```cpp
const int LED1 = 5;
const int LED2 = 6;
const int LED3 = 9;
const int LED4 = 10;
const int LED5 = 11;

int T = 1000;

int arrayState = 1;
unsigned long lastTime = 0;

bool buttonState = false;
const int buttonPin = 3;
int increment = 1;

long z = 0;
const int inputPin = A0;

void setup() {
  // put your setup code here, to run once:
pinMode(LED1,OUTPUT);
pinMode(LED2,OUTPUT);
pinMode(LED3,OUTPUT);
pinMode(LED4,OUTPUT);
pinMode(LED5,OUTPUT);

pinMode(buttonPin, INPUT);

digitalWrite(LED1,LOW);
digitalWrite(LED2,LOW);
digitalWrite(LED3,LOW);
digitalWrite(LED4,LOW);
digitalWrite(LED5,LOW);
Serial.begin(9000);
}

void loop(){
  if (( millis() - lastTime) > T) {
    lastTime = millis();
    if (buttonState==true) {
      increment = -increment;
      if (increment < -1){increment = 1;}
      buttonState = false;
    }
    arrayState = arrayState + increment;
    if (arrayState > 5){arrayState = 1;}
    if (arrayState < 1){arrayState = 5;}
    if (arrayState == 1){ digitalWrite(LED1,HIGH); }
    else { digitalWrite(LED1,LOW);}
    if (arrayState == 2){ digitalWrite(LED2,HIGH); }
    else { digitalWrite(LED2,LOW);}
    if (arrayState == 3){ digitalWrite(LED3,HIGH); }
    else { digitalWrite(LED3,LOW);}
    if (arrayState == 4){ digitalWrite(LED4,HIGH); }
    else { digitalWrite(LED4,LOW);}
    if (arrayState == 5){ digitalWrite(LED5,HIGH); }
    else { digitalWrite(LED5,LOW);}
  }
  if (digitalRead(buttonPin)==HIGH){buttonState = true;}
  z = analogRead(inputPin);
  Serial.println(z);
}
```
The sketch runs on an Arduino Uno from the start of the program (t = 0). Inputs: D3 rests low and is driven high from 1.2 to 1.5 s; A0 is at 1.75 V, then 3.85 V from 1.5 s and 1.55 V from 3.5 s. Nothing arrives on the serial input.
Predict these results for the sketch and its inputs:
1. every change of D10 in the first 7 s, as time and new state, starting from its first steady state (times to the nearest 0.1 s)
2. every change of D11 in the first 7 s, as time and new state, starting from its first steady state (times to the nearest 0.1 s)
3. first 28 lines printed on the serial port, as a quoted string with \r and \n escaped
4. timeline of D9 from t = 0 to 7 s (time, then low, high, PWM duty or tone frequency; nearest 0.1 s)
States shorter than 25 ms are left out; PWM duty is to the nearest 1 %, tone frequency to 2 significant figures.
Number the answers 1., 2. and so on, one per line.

1. 0 s low; 4 s high; 5 s low
2. 0 s low; 3 s high; 4 s low
3. "358\r\n358\r\n358\r\n358\r\n358\r\n358\r\n358\r\n358\r\n358\r\n358\r\n358\r\n358\r\n358\r\n358\r\n358\r\n358\r\n358\r\n358\r\n358\r\n358\r\n358\r\n358\r\n358\r\n358\r\n358\r\n358\r\n358\r\n358\r\n"
4. 0 s low; 5 s high; 6 s low
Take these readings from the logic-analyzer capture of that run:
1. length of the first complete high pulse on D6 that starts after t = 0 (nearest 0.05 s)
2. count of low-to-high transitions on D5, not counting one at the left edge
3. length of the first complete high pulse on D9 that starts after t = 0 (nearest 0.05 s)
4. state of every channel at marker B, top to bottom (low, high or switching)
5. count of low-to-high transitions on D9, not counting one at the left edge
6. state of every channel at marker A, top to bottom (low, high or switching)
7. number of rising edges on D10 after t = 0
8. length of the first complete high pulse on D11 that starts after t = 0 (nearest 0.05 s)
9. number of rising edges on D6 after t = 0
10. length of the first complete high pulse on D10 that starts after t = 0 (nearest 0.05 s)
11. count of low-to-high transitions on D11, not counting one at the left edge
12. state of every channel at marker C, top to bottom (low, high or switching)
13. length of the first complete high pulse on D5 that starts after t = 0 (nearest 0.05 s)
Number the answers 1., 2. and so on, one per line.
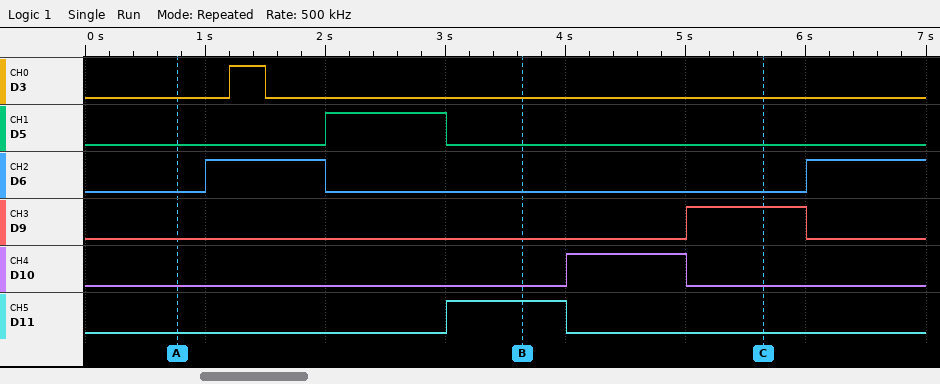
1. 1.00 s
2. 1
3. 1.00 s
4. D3 low, D5 low, D6 low, D9 low, D10 low, D11 high
5. 1
6. D3 low, D5 low, D6 low, D9 low, D10 low, D11 low
7. 1
8. 1.00 s
9. 2
10. 1.00 s
11. 1
12. D3 low, D5 low, D6 low, D9 high, D10 low, D11 low
13. 1.00 s
